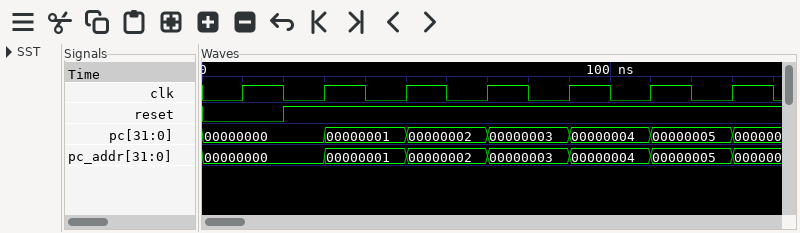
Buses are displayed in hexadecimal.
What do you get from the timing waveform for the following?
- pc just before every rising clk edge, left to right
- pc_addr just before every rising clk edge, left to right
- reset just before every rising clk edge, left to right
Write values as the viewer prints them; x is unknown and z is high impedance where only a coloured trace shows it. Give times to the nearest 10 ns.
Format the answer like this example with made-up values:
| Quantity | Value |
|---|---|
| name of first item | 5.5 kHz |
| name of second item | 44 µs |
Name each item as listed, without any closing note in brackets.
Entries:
| Quantity | Value |
|---|---|
| pc just before every rising clk edge, left to right | 00000000, 00000000, 00000001, 00000002, 00000003, 00000004, 00000005 |
| pc_addr just before every rising clk edge, left to right | 00000000, 00000000, 00000001, 00000002, 00000003, 00000004, 00000005 |
| reset just before every rising clk edge, left to right | 0 1 1 1 1 1 1 |
